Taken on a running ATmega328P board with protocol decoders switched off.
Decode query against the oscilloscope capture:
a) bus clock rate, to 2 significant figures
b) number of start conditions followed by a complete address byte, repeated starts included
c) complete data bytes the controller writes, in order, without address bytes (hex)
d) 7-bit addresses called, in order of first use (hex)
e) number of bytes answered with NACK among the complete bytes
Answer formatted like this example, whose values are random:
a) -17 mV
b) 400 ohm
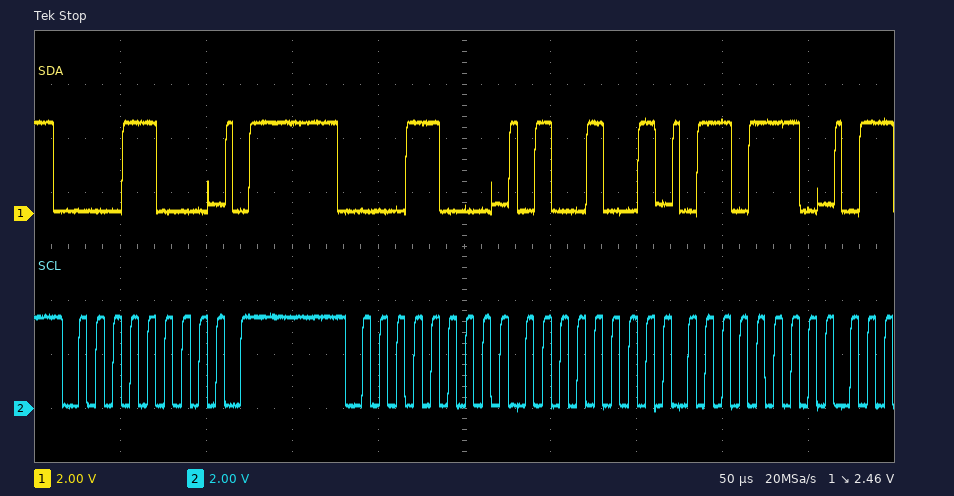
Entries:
a) 100 kHz
b) 2
c) 49 6E
d) 0x0C
e) 0
